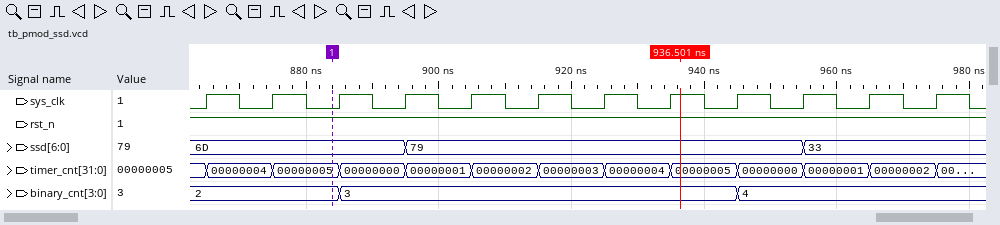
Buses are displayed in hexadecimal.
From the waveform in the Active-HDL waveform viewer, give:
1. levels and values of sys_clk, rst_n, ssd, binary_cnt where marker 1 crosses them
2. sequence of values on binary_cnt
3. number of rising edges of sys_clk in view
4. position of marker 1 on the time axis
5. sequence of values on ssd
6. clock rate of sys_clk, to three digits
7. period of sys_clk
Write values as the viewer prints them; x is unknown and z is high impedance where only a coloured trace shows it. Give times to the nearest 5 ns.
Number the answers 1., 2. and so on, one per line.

1. sys_clk=0, rst_n=1, ssd=6D, binary_cnt=2
2. 2, 3, 4
3. 12
4. 885 ns
5. 6D, 79, 33
6. 100 MHz
7. 10 ns
